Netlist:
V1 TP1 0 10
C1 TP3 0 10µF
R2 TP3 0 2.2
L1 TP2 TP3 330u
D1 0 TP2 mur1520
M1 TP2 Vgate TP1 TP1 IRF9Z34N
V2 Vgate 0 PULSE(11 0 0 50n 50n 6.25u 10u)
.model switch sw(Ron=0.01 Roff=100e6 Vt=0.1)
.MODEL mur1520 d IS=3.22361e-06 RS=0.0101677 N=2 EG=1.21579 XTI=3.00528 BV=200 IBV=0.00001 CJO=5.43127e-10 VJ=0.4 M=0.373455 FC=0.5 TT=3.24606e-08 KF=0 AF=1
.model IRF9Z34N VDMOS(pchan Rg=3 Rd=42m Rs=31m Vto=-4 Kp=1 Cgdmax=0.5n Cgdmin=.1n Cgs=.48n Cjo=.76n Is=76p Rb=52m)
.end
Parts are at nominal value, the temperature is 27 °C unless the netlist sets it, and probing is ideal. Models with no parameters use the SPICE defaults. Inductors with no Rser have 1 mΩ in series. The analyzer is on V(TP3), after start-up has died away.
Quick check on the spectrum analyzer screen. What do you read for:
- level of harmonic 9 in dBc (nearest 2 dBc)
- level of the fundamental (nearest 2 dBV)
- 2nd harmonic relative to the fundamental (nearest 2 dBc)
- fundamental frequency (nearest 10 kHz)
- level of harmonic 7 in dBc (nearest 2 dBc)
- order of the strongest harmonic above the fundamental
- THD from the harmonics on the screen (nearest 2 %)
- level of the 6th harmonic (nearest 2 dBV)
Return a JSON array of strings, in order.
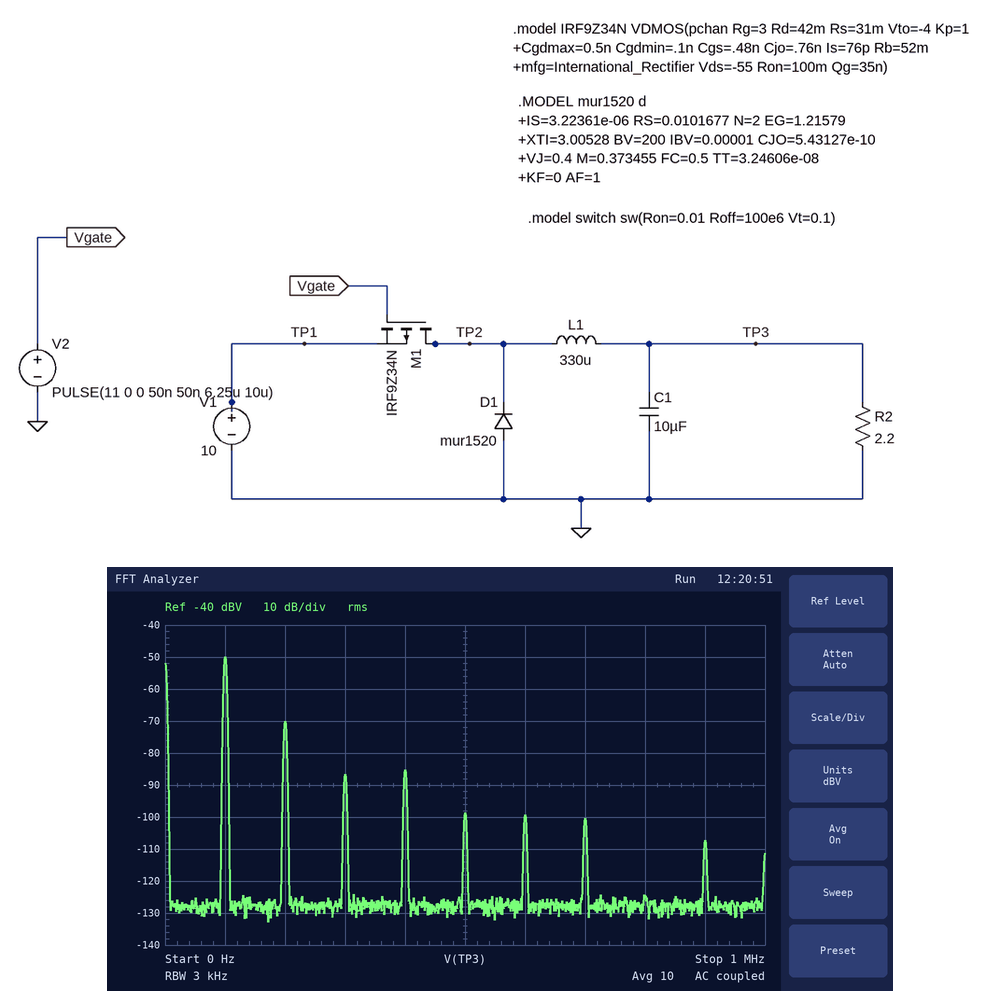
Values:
["-58 dBc", "-50 dBV", "-20 dBc", "100 kHz", "-50 dBc", "2", "10 %", "-100 dBV"]
